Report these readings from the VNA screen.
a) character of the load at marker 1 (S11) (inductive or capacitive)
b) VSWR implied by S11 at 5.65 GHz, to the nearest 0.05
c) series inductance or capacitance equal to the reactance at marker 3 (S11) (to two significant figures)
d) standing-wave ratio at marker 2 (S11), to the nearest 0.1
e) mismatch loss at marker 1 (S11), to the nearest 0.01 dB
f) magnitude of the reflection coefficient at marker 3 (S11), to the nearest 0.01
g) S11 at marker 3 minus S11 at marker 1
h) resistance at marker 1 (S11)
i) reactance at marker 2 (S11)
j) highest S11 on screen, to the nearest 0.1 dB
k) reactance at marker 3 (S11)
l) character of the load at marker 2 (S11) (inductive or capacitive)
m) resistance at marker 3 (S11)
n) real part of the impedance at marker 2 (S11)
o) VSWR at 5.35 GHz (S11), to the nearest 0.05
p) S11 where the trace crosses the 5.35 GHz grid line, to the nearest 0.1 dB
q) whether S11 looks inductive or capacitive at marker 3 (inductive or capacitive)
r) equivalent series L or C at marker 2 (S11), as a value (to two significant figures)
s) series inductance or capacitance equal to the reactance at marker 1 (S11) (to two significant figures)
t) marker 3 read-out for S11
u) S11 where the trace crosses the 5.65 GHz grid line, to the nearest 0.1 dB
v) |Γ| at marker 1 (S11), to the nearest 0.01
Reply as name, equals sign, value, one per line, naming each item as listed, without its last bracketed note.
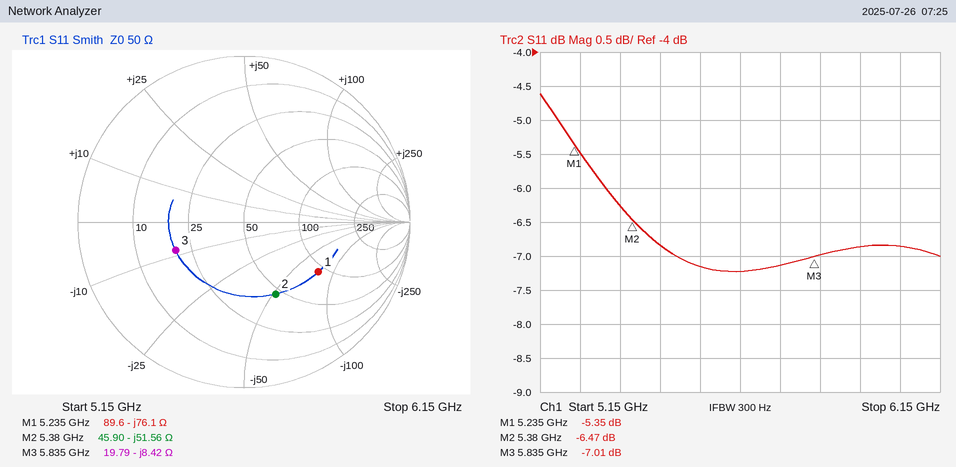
character of the load at marker 1 (S11) = capacitive
VSWR implied by S11 at 5.65 GHz, to the nearest 0.05 = 2.55
series inductance or capacitance equal to the reactance at marker 3 (S11) = 3.2 pF
standing-wave ratio at marker 2 (S11), to the nearest 0.1 = 2.8
mismatch loss at marker 1 (S11), to the nearest 0.01 dB = 1.50 dB
magnitude of the reflection coefficient at marker 3 (S11), to the nearest 0.01 = 0.45
S11 at marker 3 minus S11 at marker 1 = -1.66 dB
resistance at marker 1 = 89.6 Ω
reactance at marker 2 = -51.56 Ω
highest S11 on screen, to the nearest 0.1 dB = -4.6 dB
reactance at marker 3 = -8.42 Ω
character of the load at marker 2 (S11) = capacitive
resistance at marker 3 = 19.79 Ω
real part of the impedance at marker 2 = 45.90 Ω
VSWR at 5.35 GHz (S11), to the nearest 0.05 = 2.90
S11 where the trace crosses the 5.35 GHz grid line, to the nearest 0.1 dB = -6.3 dB
whether S11 looks inductive or capacitive at marker 3 = capacitive
equivalent series L or C at marker 2 (S11), as a value = 570 fF
series inductance or capacitance equal to the reactance at marker 1 (S11) = 400 fF
marker 3 read-out for S11 = -7.01 dB
S11 where the trace crosses the 5.65 GHz grid line, to the nearest 0.1 dB = -7.2 dB
|Γ| at marker 1 (S11), to the nearest 0.01 = 0.54
